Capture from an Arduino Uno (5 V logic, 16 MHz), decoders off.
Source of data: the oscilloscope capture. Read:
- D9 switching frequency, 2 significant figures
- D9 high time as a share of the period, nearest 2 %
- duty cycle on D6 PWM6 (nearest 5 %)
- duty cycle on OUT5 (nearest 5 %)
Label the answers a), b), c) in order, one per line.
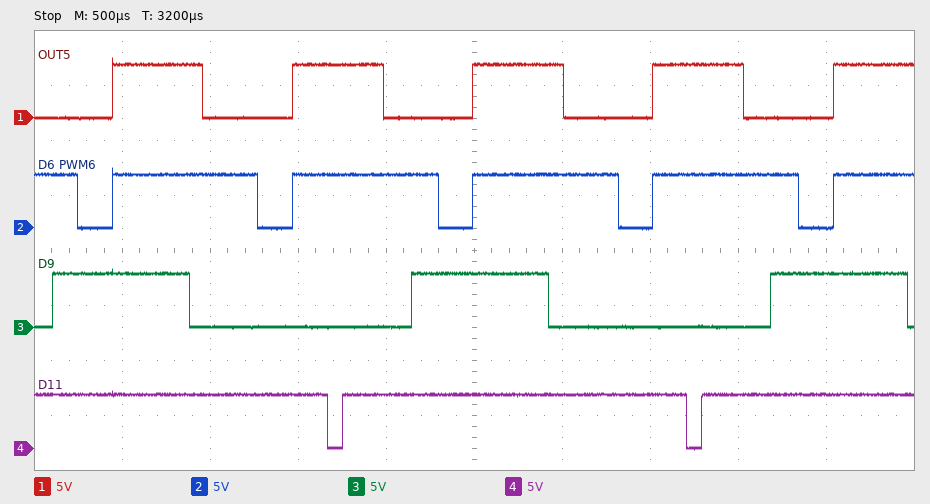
a) 490 Hz
b) 38 %
c) 80 %
d) 50 %
